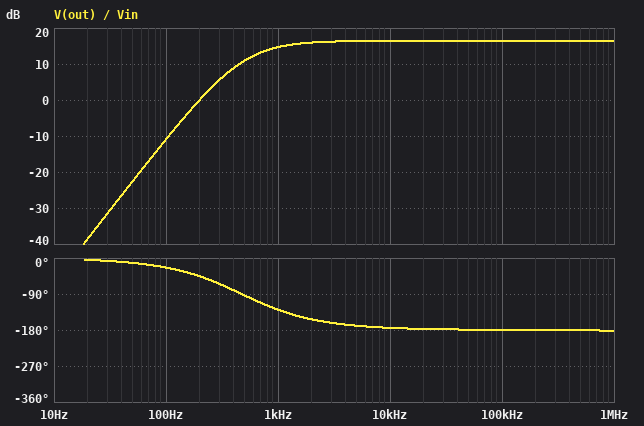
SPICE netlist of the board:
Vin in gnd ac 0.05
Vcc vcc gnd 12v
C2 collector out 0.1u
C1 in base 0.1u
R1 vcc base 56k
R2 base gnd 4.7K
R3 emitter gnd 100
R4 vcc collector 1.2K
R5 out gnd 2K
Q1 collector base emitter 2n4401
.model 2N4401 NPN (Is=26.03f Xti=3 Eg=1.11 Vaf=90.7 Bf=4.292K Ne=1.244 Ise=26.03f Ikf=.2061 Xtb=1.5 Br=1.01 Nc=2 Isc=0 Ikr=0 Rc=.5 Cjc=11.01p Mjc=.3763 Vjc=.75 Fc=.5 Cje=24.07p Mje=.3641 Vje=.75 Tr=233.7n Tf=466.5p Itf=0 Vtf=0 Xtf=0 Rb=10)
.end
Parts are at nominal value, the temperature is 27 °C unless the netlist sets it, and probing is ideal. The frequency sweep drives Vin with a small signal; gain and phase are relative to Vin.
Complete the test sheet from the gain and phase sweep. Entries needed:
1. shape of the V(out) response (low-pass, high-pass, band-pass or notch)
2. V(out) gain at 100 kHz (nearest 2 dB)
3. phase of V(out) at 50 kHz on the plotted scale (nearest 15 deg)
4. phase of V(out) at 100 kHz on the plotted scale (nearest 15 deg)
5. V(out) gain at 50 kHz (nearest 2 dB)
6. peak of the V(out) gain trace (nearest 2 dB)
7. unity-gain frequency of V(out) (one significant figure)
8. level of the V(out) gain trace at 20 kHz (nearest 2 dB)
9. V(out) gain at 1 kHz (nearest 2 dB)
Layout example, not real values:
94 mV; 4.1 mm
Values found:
high-pass; 16 dB; -180 deg; -180 deg; 16 dB; 16 dB; 200 Hz; 16 dB; 14 dB
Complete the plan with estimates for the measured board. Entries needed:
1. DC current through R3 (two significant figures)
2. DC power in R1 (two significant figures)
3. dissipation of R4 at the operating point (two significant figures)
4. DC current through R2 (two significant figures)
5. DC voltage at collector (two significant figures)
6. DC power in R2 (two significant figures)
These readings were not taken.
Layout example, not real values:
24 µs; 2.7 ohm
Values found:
2.2 mA; 2.2 mW; 5.5 mW; 180 µA; 9.4 V; 160 µW
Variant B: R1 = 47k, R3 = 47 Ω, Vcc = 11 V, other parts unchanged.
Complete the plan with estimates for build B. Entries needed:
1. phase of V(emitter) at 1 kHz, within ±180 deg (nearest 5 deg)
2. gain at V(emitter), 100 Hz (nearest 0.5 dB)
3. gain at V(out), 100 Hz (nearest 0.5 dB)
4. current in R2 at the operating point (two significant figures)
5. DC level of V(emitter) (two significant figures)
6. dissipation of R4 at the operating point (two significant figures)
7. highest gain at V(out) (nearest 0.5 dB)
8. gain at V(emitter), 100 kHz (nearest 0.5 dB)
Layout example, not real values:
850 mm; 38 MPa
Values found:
30 deg; -16.0 dB; -6.0 dB; 190 µA; 210 mV; 24 mW; 23.0 dB; -1.0 dB
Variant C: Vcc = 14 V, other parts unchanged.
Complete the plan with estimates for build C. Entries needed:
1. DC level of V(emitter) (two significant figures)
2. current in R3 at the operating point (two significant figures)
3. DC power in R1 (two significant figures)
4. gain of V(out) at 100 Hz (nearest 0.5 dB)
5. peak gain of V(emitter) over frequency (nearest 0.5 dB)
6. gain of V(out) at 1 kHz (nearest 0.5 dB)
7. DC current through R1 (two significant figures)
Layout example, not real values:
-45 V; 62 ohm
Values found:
330 mV; 3.3 mA; 3.0 mW; -10.5 dB; -0.5 dB; 15.0 dB; 230 µA
